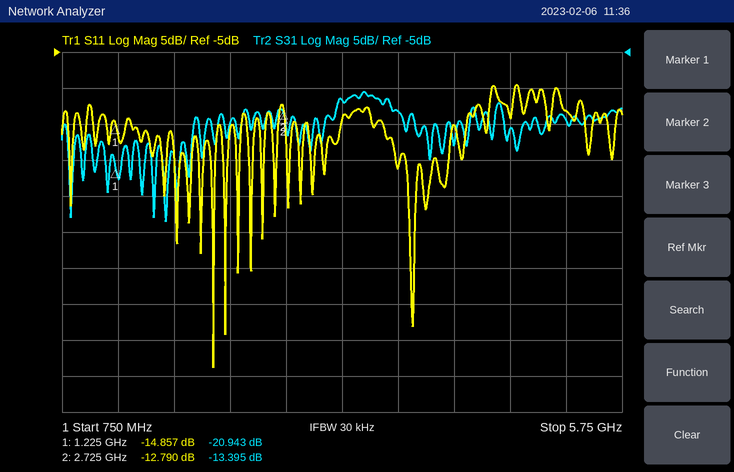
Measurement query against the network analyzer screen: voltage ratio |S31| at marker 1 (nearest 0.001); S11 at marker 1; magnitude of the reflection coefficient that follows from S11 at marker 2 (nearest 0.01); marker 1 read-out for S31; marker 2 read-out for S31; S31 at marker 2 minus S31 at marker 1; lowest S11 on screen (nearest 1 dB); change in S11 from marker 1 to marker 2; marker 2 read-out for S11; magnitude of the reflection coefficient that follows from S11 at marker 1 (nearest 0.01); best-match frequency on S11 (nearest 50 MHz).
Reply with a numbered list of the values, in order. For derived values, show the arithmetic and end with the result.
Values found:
1. 10^(-20.943/20) ≈ 0.090
2. -14.857 dB
3. 10^(-12.79/20) ≈ 0.23
4. -20.943 dB
5. -13.395 dB
6. -13.395 − (-20.943) = 7.548 dB
7. -49 dB
8. -12.79 − (-14.857) = 2.067 dB
9. -12.790 dB
10. 10^(-14.857/20) ≈ 0.18
11. 2.10 GHz
